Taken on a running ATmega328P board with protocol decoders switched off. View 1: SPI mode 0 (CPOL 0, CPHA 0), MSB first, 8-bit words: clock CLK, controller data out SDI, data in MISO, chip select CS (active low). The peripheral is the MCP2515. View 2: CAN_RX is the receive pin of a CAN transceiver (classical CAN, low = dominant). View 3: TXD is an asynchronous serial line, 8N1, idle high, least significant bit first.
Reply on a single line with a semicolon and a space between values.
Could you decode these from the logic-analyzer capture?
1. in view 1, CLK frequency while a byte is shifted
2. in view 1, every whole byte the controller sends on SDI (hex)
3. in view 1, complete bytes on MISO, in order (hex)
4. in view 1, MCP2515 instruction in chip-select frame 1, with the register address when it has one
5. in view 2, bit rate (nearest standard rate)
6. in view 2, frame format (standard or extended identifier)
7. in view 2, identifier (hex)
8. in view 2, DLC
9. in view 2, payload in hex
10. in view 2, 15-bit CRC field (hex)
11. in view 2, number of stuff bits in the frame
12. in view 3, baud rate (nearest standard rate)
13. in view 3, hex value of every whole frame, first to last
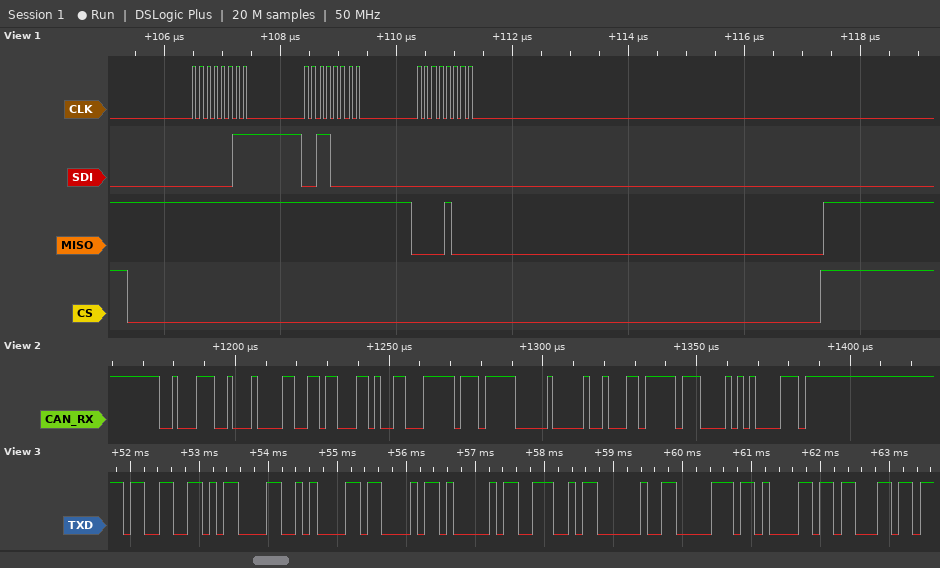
8 MHz; 0x03 0x30 0x00; 0xFF 0xFF 0x08; READ 0x30; 500 kbit/s; standard; 0x239; 8; 66 C6 98 FF 7C 00 46 FF; 0x0543; 5; 9600 baud; 33 0D 0A 43 41 4E 20 70 61 63
